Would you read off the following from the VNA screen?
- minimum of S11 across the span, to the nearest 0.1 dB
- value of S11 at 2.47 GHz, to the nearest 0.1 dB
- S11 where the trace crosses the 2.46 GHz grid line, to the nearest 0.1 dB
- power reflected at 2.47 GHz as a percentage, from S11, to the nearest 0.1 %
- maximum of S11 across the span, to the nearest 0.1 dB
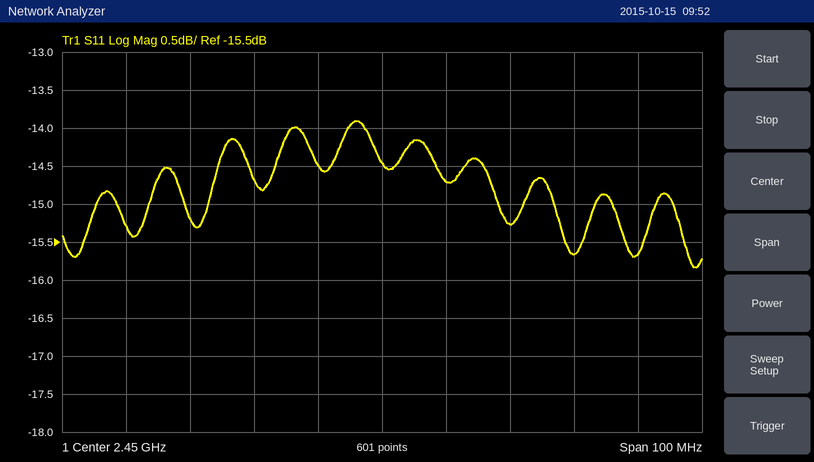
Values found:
-15.8 dB
-15.3 dB
-14.7 dB
3.0 %
-13.9 dB
